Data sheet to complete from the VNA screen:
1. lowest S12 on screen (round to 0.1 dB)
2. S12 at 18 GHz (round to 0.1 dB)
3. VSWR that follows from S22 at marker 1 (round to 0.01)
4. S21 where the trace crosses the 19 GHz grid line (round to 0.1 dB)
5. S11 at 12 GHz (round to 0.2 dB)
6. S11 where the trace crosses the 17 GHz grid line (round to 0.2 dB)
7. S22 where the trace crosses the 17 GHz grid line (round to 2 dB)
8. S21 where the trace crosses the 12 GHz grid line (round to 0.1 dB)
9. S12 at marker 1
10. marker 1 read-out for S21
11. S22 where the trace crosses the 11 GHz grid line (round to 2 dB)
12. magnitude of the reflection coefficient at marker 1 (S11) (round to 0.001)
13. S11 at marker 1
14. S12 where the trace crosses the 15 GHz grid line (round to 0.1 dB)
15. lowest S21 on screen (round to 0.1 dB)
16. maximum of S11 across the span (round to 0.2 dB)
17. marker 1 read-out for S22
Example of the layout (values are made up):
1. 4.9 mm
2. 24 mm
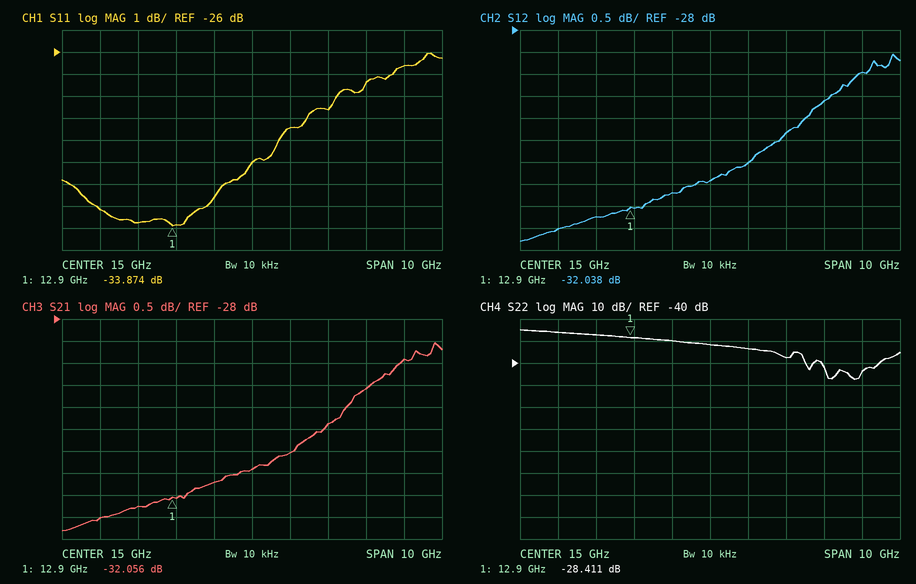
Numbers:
1. -32.8 dB
2. -29.6 dB
3. 1.08
4. -28.9 dB
5. -33.8 dB
6. -28.6 dB
7. -38 dB
8. -32.3 dB
9. -32.038 dB
10. -32.056 dB
11. -26 dB
12. 0.020
13. -33.874 dB
14. -31.4 dB
15. -32.8 dB
16. -26.0 dB
17. -28.411 dB
